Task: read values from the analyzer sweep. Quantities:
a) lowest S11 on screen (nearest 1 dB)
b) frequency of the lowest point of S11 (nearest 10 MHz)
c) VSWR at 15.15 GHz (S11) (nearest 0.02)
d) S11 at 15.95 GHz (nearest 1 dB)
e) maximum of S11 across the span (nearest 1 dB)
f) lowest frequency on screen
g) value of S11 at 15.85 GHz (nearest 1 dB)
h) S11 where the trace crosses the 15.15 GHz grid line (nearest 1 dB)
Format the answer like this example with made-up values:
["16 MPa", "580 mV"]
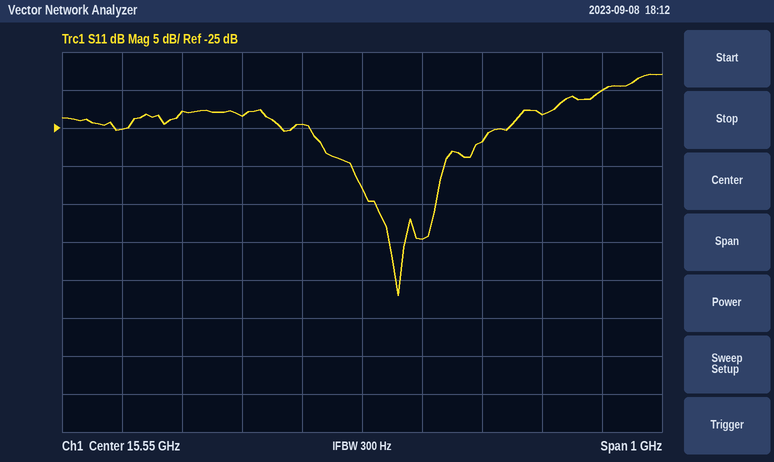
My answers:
["-47 dB", "15.61 GHz", "1.12", "-20 dB", "-18 dB", "15.05 GHz", "-23 dB", "-25 dB"]
